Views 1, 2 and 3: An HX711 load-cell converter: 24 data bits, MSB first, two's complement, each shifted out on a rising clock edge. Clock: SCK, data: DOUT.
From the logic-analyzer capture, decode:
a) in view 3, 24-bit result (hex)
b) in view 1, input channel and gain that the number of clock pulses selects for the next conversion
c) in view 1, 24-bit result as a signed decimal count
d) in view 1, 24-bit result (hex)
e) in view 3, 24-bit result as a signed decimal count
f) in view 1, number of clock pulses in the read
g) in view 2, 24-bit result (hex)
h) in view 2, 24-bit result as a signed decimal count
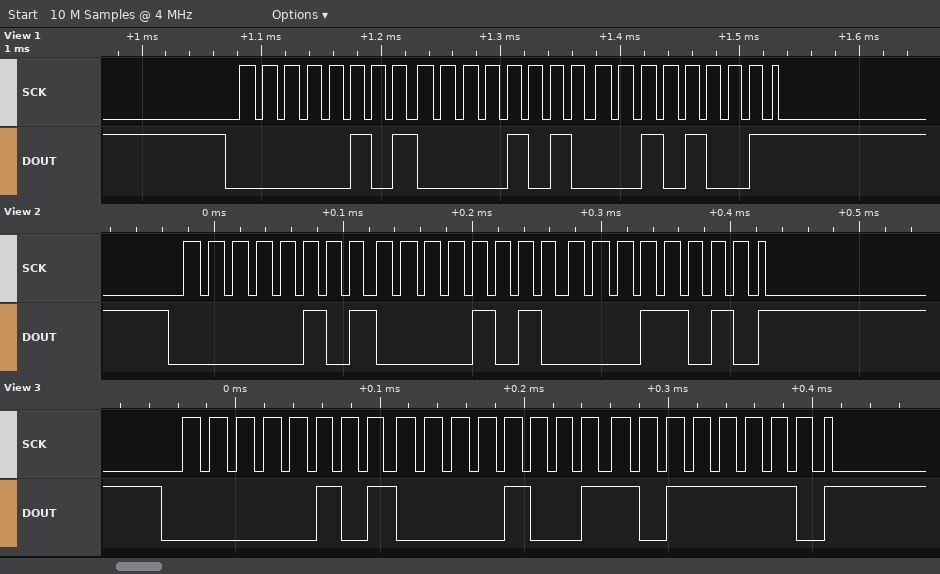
0x0509BE
channel A, gain 128
330281
0x050A29
330174
25
0x050A1A
330266
